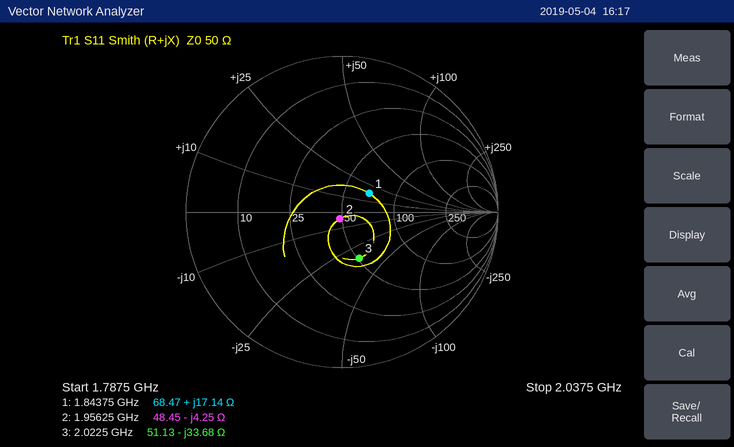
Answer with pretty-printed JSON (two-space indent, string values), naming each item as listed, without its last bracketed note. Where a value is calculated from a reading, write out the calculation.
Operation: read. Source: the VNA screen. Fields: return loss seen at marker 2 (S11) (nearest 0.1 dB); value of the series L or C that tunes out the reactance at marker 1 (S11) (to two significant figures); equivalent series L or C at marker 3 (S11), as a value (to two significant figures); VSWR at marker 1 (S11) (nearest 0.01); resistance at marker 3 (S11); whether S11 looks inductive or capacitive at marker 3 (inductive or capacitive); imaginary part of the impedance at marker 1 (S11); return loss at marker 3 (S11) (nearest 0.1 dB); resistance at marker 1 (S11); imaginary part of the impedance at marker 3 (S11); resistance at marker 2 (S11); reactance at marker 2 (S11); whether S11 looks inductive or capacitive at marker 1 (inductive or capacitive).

{
  "return loss seen at marker 2 (S11)": "26.8 dB",
  "value of the series L or C that tunes out the reactance at marker 1 (S11)": "C = 1/(2π × 1.84375 GHz × 17.14 Ω) ≈ 5.0 pF",
  "equivalent series L or C at marker 3 (S11), as a value": "C = 1/(2π × 2.0225 GHz × 33.68 Ω) ≈ 2.3 pF",
  "VSWR at marker 1 (S11)": "1.53",
  "resistance at marker 3": "51.13 Ω",
  "whether S11 looks inductive or capacitive at marker 3": "capacitive",
  "imaginary part of the impedance at marker 1": "+17.14 Ω",
  "return loss at marker 3 (S11)": "10.0 dB",
  "resistance at marker 1": "68.47 Ω",
  "imaginary part of the impedance at marker 3": "-33.68 Ω",
  "resistance at marker 2": "48.45 Ω",
  "reactance at marker 2": "-4.25 Ω",
  "whether S11 looks inductive or capacitive at marker 1": "inductive"
}
